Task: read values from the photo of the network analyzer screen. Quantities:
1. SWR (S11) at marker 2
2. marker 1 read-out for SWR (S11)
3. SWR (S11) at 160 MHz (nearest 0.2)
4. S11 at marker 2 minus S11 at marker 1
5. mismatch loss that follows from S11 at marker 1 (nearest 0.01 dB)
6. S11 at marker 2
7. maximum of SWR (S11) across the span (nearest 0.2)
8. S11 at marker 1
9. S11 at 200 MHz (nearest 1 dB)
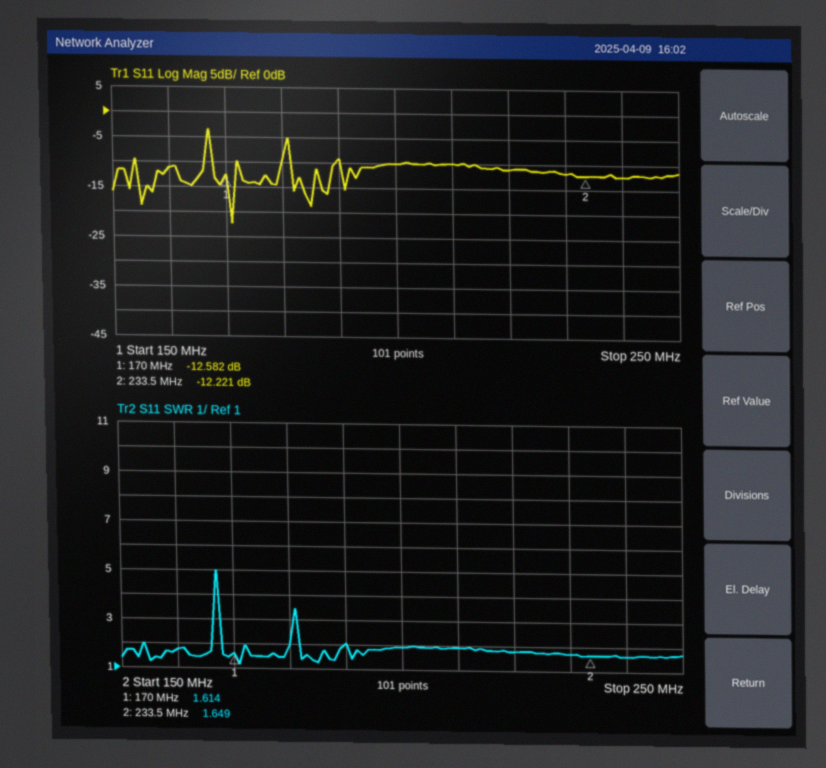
1.649
1.614
1.8
0.361 dB
0.25 dB
-12.221 dB
5.0
-12.582 dB
-10 dB
